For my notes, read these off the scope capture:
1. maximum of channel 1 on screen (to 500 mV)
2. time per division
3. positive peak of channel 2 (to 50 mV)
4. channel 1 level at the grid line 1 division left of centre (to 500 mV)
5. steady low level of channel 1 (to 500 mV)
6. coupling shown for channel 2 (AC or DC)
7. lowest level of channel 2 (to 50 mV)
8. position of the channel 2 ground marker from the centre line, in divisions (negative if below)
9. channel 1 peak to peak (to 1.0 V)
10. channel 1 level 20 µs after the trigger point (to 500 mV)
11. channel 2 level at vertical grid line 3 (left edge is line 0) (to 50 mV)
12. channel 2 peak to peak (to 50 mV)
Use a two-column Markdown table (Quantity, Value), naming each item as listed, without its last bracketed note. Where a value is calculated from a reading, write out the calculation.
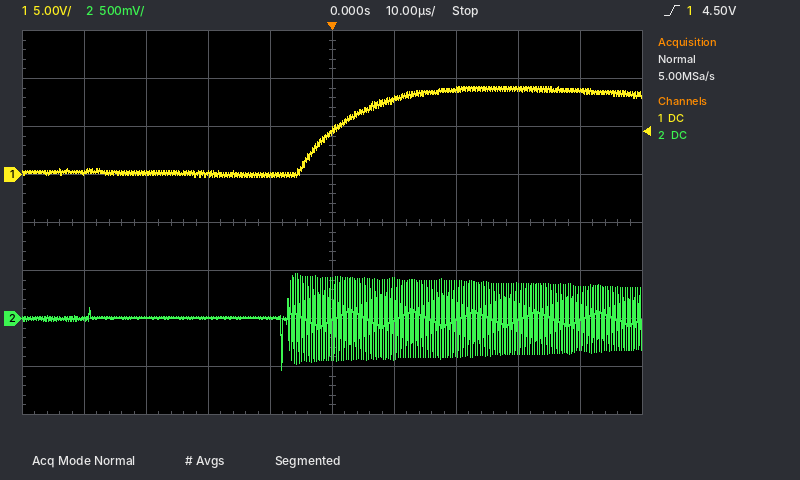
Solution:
| Quantity | Value |
|---|---|
| maximum of channel 1 on screen | 9.0 V |
| time per division | 10 µs |
| positive peak of channel 2 | 450 mV |
| channel 1 level at the grid line 1 division left of centre | 0.0 V |
| steady low level of channel 1 | 0.0 V |
| coupling shown for channel 2 | DC |
| lowest level of channel 2 | -550 mV |
| position of the channel 2 ground marker from the centre line, in divisions | -2.0 div |
| channel 1 peak to peak | 9.0 V |
| channel 1 level 20 µs after the trigger point | 9.0 V |
| channel 2 level at vertical grid line 3 (left edge is line 0) | 0 mV |
| channel 2 peak to peak | 450 mV − (-550 mV) = 1.00 V |
